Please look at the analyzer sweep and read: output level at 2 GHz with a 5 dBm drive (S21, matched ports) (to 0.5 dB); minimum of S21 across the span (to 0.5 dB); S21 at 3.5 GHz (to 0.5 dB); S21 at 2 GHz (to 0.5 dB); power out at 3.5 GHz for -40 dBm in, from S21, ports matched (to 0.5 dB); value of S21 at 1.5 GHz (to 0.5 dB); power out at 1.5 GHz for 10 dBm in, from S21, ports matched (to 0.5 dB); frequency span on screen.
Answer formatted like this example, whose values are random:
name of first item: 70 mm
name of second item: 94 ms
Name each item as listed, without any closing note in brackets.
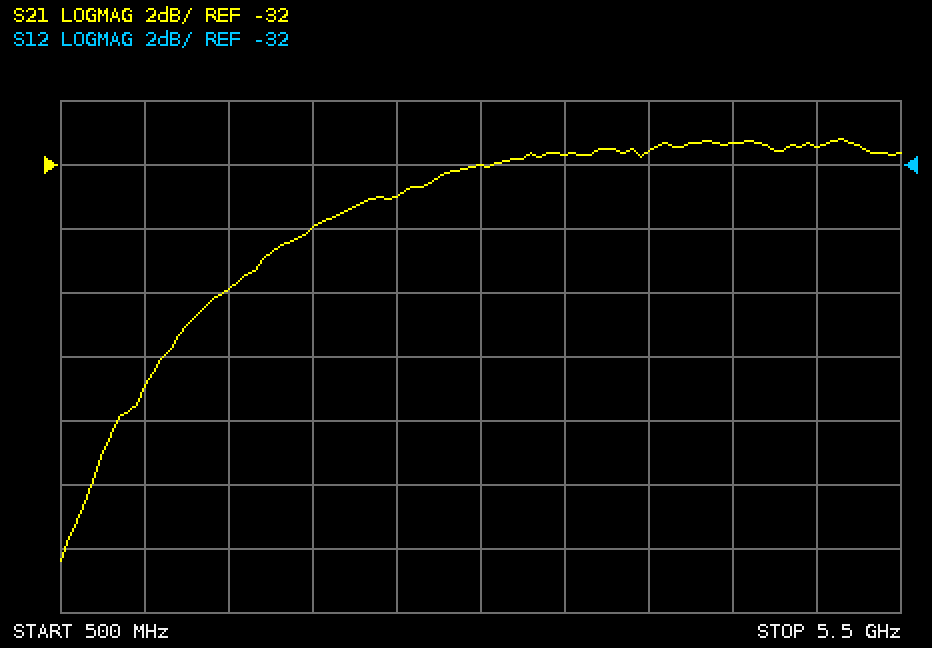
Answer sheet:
output level at 2 GHz with a 5 dBm drive (S21, matched ports): -29.0 dBm
minimum of S21 across the span: -44.5 dB
S21 at 3.5 GHz: -31.5 dB
S21 at 2 GHz: -34.0 dB
power out at 3.5 GHz for -40 dBm in, from S21, ports matched: -71.5 dBm
value of S21 at 1.5 GHz: -36.0 dB
power out at 1.5 GHz for 10 dBm in, from S21, ports matched: -26.0 dBm
frequency span on screen: 5 GHz
